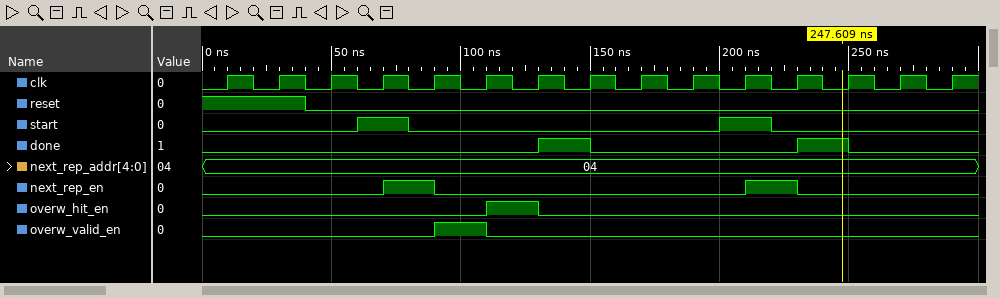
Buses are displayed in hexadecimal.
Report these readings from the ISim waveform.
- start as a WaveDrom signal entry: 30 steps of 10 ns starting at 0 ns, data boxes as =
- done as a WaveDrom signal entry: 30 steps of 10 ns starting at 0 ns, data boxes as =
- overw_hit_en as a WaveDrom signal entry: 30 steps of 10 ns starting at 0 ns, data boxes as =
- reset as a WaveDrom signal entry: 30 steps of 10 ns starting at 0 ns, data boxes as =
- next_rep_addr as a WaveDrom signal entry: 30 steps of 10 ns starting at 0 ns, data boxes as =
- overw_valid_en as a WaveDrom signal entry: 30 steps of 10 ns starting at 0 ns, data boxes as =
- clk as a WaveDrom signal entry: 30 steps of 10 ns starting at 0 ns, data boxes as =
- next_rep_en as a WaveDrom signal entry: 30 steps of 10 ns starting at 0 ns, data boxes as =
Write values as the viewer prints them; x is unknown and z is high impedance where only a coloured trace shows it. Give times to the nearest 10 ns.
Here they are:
{name: 'start', wave: '0.....1.0...........1.0.......'}
{name: 'done', wave: '0............1.0.......1.0....'}
{name: 'overw_hit_en', wave: '0..........1.0................'}
{name: 'reset', wave: '1...0.........................'}
{name: 'next_rep_addr', wave: '=.............................', data: '04'}
{name: 'overw_valid_en', wave: '0........1.0..................'}
{name: 'clk', wave: '010101010101010101010101010101'}
{name: 'next_rep_en', wave: '0......1.0...........1.0......'}
